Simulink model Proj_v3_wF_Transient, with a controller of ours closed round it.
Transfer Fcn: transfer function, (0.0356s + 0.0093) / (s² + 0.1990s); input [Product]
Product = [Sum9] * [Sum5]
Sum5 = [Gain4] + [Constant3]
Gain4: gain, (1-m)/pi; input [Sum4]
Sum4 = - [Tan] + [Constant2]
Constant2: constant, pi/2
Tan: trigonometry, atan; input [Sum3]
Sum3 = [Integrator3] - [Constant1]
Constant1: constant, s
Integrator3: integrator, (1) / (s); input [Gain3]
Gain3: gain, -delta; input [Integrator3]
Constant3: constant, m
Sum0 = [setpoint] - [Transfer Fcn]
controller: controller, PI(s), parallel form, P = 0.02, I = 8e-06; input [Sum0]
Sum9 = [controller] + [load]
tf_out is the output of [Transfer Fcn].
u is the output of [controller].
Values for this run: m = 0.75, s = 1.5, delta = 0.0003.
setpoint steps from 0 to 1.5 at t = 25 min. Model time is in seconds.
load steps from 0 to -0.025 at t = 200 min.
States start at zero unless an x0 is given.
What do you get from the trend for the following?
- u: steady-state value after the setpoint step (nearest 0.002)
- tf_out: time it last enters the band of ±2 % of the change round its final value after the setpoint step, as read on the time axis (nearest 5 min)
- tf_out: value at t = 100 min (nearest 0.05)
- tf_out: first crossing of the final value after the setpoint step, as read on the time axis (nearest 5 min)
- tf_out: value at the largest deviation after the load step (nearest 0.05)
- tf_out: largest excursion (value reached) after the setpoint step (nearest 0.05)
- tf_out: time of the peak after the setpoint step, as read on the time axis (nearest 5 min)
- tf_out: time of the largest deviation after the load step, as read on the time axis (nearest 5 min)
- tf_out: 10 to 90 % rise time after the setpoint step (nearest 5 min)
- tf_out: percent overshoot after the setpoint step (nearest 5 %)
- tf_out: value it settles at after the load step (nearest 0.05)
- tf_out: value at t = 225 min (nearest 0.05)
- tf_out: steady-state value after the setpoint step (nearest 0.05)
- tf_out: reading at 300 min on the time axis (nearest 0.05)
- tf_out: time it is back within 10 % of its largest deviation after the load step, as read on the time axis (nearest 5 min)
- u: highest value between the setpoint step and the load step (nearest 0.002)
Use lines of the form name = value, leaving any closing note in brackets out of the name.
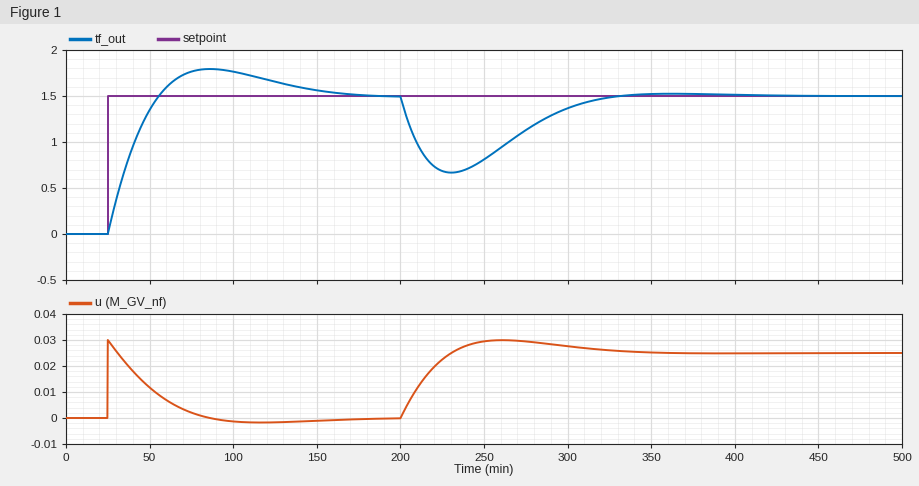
u: steady-state value after the setpoint step = 0.000
tf_out: time it last enters the band of ±2 % of the change round its final value after the setpoint step, as read on the time axis = 165 min
tf_out: value at t = 100 min = 1.75
tf_out: first crossing of the final value after the setpoint step, as read on the time axis = 55 min
tf_out: value at the largest deviation after the load step = 0.65
tf_out: largest excursion (value reached) after the setpoint step = 1.80
tf_out: time of the peak after the setpoint step, as read on the time axis = 85 min
tf_out: time of the largest deviation after the load step, as read on the time axis = 230 min
tf_out: 10 to 90 % rise time after the setpoint step = 25 min
tf_out: percent overshoot after the setpoint step = 20 %
tf_out: value it settles at after the load step = 1.50
tf_out: value at t = 225 min = 0.70
tf_out: steady-state value after the setpoint step = 1.50
tf_out: reading at 300 min on the time axis = 1.35
tf_out: time it is back within 10 % of its largest deviation after the load step, as read on the time axis = 310 min
u: highest value between the setpoint step and the load step = 0.030
